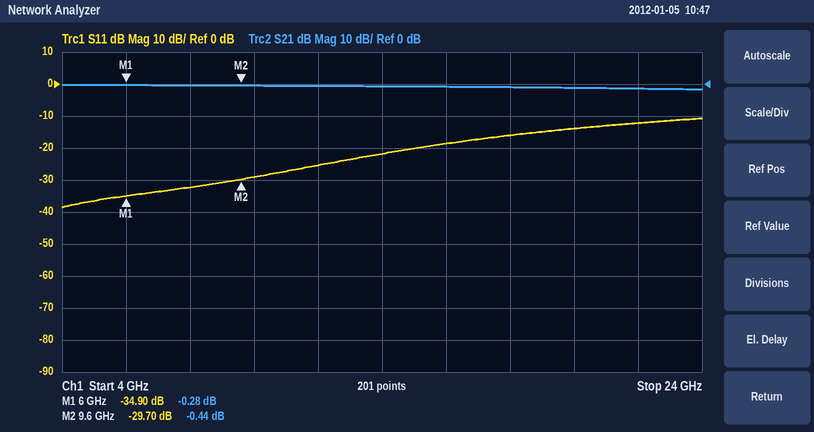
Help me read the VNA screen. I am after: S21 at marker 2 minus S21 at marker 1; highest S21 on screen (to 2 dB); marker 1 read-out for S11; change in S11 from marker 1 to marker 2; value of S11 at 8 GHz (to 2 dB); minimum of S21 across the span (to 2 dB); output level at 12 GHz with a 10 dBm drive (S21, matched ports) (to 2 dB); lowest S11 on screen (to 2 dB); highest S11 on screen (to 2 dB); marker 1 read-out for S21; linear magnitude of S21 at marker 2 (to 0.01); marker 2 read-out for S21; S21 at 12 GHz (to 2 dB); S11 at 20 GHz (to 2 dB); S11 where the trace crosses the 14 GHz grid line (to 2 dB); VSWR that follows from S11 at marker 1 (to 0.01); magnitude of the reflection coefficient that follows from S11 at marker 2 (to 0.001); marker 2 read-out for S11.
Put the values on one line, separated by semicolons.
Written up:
-0.16 dB; 0 dB; -34.90 dB; 5.20 dB; -32 dB; -2 dB; 10 dBm; -38 dB; -10 dB; -0.28 dB; 0.95; -0.44 dB; 0 dB; -14 dB; -22 dB; 1.04; 0.033; -29.70 dB
